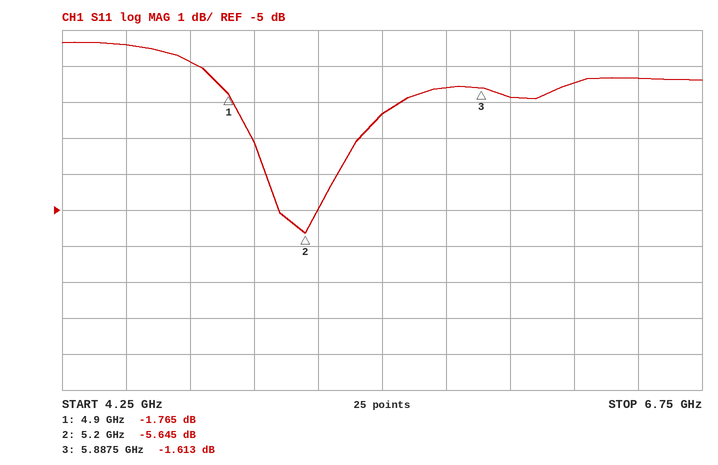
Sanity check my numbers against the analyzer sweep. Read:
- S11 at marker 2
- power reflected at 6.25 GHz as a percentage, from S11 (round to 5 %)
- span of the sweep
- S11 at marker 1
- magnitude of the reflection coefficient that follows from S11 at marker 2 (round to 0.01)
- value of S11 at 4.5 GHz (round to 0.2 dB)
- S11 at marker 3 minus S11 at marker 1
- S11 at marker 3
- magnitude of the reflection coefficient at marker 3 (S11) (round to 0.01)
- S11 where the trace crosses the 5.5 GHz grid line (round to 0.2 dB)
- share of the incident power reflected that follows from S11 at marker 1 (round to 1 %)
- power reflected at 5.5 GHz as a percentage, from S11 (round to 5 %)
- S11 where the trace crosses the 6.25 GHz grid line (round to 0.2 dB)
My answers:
-5.645 dB
70 %
2.5 GHz
-1.765 dB
0.52
-0.4 dB
0.152 dB
-1.613 dB
0.83
-2.4 dB
67 %
60 %
-1.4 dB
